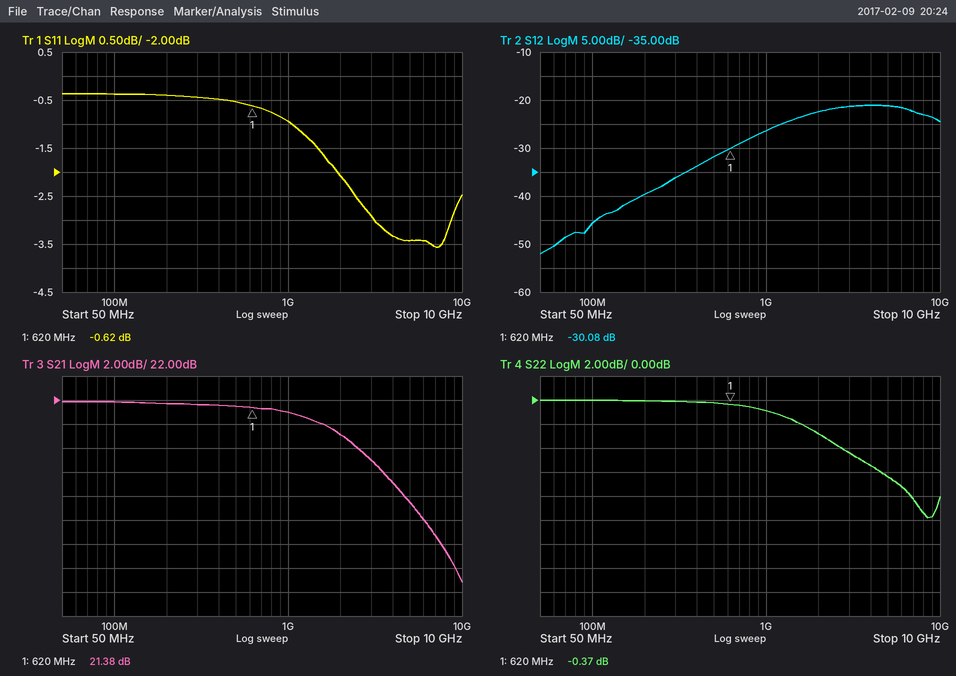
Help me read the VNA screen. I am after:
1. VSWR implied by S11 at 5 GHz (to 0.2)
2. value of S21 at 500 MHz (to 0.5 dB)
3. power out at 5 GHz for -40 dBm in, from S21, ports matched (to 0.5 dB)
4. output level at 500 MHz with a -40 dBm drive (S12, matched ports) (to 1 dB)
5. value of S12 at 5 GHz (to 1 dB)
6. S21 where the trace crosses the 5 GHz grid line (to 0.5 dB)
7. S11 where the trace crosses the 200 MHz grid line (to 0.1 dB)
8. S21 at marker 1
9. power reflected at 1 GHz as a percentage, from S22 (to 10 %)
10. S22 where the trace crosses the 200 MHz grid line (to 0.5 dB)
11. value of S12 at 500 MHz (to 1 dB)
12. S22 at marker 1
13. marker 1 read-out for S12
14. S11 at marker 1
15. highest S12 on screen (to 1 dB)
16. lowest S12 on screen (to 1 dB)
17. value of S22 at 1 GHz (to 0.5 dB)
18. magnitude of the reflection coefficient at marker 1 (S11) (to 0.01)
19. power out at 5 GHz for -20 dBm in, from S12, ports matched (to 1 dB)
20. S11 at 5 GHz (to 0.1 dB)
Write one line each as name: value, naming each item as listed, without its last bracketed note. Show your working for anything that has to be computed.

VSWR implied by S11 at 5 GHz: |Γ| = 10^(-3.4/20) = 0.6761; VSWR = (1 + 0.6761)/(1 − 0.6761) ≈ 5.2
value of S21 at 500 MHz: 21.5 dB
power out at 5 GHz for -40 dBm in, from S21, ports matched: -40 dBm + (13.5 dB) = -26.5 dBm
output level at 500 MHz with a -40 dBm drive (S12, matched ports): -40 dBm + (-32 dB) = -72 dBm
value of S12 at 5 GHz: -21 dB
S21 where the trace crosses the 5 GHz grid line: 13.5 dB
S11 where the trace crosses the 200 MHz grid line: -0.4 dB
S21 at marker 1: 21.38 dB
power reflected at 1 GHz as a percentage, from S22: 10^(-1/10) ≈ 79.4 %, so 80 % to the nearest 10 %
S22 where the trace crosses the 200 MHz grid line: 0.0 dB
value of S12 at 500 MHz: -32 dB
S22 at marker 1: -0.37 dB
marker 1 read-out for S12: -30.08 dB
S11 at marker 1: -0.62 dB
highest S12 on screen: -21 dB
lowest S12 on screen: -52 dB
value of S22 at 1 GHz: -1.0 dB
magnitude of the reflection coefficient at marker 1 (S11): 10^(-0.62/20) ≈ 0.93
power out at 5 GHz for -20 dBm in, from S12, ports matched: -20 dBm + (-21 dB) = -41 dBm
S11 at 5 GHz: -3.4 dB
